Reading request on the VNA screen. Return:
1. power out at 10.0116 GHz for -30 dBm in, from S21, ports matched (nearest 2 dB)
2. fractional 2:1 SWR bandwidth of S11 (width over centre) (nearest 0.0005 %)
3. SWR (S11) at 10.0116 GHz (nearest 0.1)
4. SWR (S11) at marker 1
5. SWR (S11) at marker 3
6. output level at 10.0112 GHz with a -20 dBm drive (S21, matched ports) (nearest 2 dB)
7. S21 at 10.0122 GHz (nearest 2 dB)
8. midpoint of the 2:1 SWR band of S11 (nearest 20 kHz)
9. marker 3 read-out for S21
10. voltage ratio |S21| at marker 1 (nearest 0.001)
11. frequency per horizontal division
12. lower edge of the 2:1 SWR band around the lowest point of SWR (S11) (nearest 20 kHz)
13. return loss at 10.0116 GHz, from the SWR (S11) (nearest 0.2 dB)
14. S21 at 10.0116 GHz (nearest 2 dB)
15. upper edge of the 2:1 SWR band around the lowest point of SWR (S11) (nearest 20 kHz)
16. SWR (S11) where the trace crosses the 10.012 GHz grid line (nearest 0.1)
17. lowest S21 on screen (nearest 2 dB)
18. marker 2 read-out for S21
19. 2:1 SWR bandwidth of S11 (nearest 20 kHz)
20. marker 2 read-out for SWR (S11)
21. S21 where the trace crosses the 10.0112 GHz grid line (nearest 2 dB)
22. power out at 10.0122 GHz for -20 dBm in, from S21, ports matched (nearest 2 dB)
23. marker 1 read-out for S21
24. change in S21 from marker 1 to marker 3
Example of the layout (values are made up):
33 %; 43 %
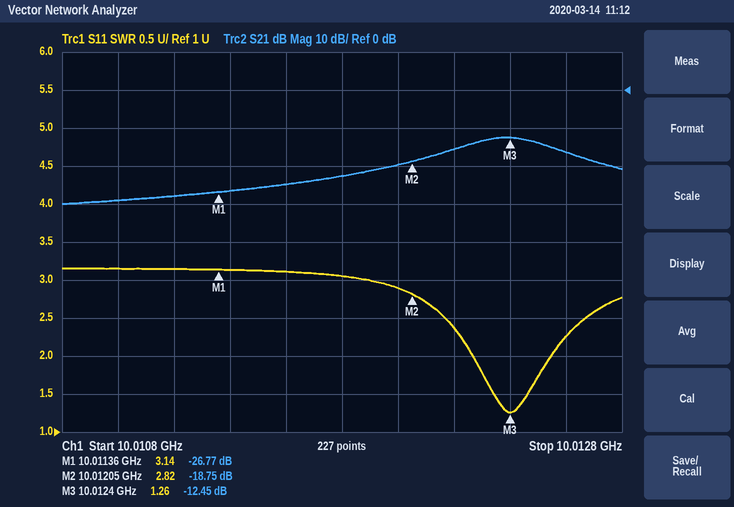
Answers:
-54 dBm; 0.0030 %; 3.1; 3.14; 1.26; -48 dBm; -16 dB; 10.01240 GHz; -12.45 dB; 0.046; 200 kHz; 10.01226 GHz; 5.8 dB; -24 dB; 10.01254 GHz; 2.9; -30 dB; -18.75 dB; 280 kHz; 2.82; -28 dB; -36 dBm; -26.77 dB; 14.32 dB
